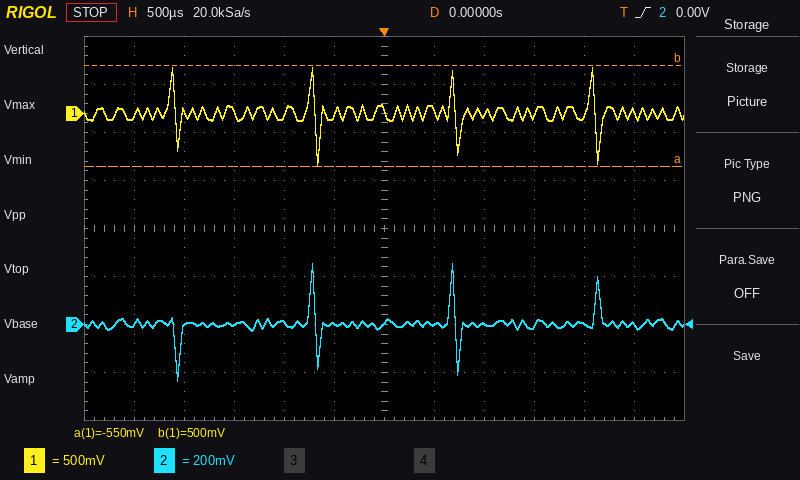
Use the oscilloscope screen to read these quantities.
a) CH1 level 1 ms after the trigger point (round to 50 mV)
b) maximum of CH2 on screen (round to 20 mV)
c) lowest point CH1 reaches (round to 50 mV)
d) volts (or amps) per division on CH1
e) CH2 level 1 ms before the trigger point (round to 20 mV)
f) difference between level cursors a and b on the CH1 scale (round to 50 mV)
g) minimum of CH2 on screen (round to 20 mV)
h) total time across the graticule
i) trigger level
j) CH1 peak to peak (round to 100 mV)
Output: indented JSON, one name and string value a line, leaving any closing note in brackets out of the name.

{
  "CH1 level 1 ms after the trigger point": "0 mV",
  "maximum of CH2 on screen": "260 mV",
  "lowest point CH1 reaches": "-550 mV",
  "volts (or amps) per division on CH1": "500 mV",
  "CH2 level 1 ms before the trigger point": "0 mV",
  "difference between level cursors a and b on the CH1 scale": "1.05 V",
  "minimum of CH2 on screen": "-240 mV",
  "total time across the graticule": "6 ms",
  "trigger level": "0.00 V",
  "CH1 peak to peak": "1.00 V"
}
